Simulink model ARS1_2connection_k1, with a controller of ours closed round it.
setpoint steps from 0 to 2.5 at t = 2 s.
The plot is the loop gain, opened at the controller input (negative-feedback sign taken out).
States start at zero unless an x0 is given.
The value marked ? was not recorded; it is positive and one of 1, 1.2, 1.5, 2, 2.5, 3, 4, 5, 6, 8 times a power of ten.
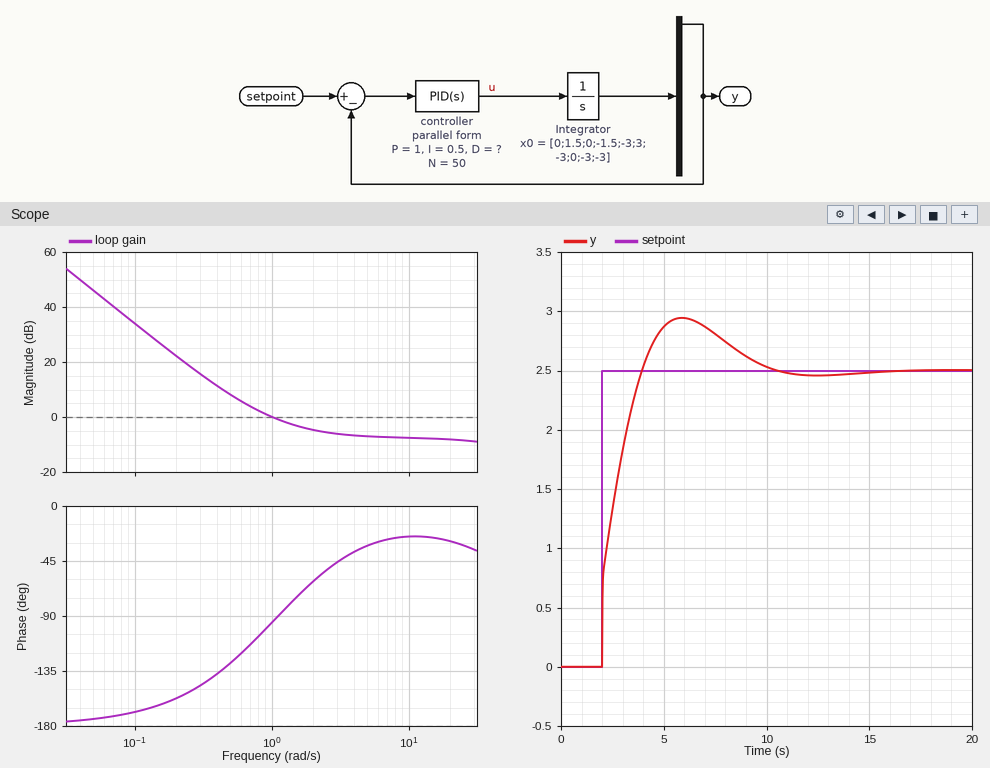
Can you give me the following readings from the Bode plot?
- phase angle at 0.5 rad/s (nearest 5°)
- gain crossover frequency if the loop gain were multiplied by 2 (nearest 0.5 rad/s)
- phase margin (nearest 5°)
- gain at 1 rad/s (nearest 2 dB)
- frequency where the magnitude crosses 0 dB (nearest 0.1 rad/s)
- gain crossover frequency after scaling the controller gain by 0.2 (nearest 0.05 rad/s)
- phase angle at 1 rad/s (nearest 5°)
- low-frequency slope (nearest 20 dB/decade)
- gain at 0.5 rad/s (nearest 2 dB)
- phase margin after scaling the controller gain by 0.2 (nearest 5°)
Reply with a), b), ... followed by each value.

a) -130°
b) 3.0 rad/s
c) 85°
d) 0 dB
e) 1.0 rad/s
f) 0.35 rad/s
g) -95°
h) -40 dB/decade
i) 8 dB
j) 35°
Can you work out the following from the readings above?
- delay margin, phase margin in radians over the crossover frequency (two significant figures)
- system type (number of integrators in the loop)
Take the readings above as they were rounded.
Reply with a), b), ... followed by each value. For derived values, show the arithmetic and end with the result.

a) 85 × π / 180 / 1 = 1.5 s
b) 2
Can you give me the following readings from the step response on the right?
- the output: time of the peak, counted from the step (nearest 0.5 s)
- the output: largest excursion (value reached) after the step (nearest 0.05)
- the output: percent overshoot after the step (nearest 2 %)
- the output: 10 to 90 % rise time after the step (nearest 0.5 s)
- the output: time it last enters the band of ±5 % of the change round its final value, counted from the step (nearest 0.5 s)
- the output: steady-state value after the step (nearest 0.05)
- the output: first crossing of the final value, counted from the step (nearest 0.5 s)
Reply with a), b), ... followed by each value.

a) 4.0 s
b) 2.95
c) 18 %
d) 1.5 s
e) 7.0 s
f) 2.50
g) 2.0 s
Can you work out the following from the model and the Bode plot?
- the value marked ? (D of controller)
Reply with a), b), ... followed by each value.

a) 0.4
